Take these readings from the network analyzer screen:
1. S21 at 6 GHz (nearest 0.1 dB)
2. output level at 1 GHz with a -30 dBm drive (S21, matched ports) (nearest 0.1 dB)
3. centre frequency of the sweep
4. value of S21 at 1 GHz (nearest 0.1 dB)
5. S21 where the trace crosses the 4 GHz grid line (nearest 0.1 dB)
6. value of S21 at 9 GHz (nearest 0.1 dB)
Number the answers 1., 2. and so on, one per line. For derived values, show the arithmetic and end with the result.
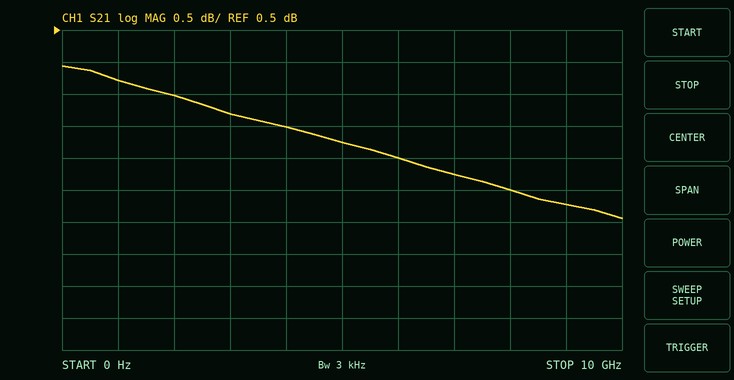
1. -1.5 dB
2. -30 dBm + (-0.3 dB) = -30.3 dBm
3. 5 GHz
4. -0.3 dB
5. -1.0 dB
6. -2.2 dB
